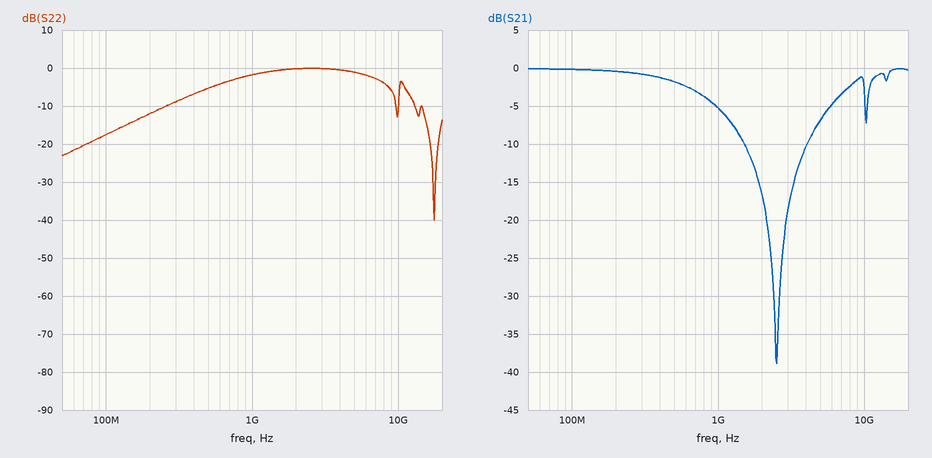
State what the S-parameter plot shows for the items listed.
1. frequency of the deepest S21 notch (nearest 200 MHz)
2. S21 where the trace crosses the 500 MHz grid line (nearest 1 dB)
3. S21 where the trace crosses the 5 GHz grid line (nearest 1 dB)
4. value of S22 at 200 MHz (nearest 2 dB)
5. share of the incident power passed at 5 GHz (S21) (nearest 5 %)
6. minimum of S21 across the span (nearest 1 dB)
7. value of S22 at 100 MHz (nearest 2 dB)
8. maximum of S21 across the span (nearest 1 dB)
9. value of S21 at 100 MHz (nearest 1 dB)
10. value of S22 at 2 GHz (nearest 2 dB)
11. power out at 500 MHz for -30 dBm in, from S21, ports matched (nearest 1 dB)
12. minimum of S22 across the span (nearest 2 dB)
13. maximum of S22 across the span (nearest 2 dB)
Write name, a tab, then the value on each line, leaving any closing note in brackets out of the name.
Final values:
frequency of the deepest S21 notch	2.6 GHz
S21 where the trace crosses the 500 MHz grid line	-2 dB
S21 where the trace crosses the 5 GHz grid line	-7 dB
value of S22 at 200 MHz	-12 dB
share of the incident power passed at 5 GHz (S21)	20 %
minimum of S21 across the span	-39 dB
value of S22 at 100 MHz	-18 dB
maximum of S21 across the span	0 dB
value of S21 at 100 MHz	0 dB
value of S22 at 2 GHz	0 dB
power out at 500 MHz for -30 dBm in, from S21, ports matched	-32 dBm
minimum of S22 across the span	-40 dB
maximum of S22 across the span	0 dB
